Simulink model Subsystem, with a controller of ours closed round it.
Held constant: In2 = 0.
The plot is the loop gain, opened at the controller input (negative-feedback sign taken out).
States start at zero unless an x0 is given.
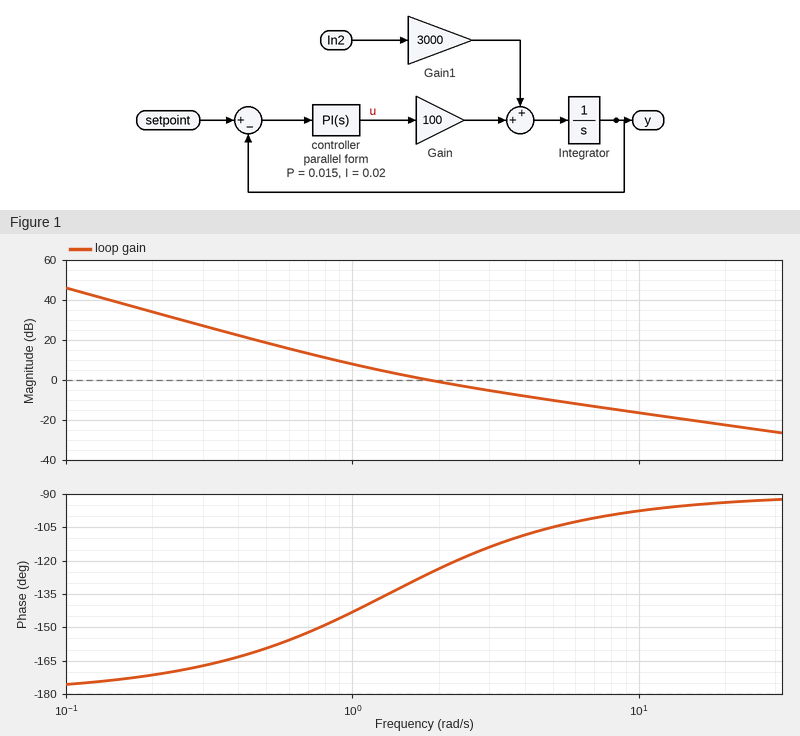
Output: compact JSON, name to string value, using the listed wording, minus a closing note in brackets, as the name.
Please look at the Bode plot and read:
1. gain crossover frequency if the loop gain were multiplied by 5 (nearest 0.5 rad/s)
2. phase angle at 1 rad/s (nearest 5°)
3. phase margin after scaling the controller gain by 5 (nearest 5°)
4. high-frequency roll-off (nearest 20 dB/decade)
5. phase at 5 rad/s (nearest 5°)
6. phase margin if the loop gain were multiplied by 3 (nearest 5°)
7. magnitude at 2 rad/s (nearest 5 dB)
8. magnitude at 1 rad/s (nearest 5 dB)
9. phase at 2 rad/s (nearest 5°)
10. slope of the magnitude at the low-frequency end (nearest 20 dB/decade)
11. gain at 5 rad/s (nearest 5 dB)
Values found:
{"gain crossover frequency if the loop gain were multiplied by 5": "7.5 rad/s", "phase angle at 1 rad/s": "-145°", "phase margin after scaling the controller gain by 5": "80°", "high-frequency roll-off": "-20 dB/decade", "phase at 5 rad/s": "-105°", "phase margin if the loop gain were multiplied by 3": "75°", "magnitude at 2 rad/s": "0 dB", "magnitude at 1 rad/s": "10 dB", "phase at 2 rad/s": "-125°", "slope of the magnitude at the low-frequency end": "-40 dB/decade", "gain at 5 rad/s": "-10 dB"}
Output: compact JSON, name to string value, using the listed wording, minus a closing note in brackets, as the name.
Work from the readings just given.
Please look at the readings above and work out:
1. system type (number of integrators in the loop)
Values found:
{"system type": "2"}
